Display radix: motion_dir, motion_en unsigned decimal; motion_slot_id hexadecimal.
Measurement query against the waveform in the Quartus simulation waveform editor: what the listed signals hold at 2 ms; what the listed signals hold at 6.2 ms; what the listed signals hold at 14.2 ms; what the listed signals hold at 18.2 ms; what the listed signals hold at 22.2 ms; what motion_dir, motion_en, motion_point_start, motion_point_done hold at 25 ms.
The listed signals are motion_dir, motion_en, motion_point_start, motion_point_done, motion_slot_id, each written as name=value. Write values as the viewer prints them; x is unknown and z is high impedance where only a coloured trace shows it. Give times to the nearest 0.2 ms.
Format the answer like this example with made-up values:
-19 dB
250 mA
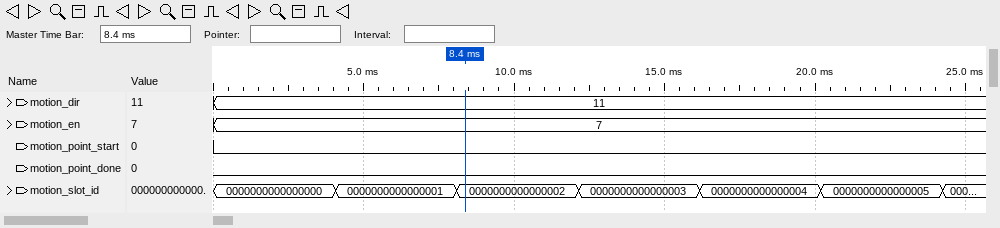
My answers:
motion_dir=11, motion_en=7, motion_point_start=0, motion_point_done=0, motion_slot_id=0000000000000000
motion_dir=11, motion_en=7, motion_point_start=0, motion_point_done=0, motion_slot_id=0000000000000001
motion_dir=11, motion_en=7, motion_point_start=0, motion_point_done=0, motion_slot_id=0000000000000003
motion_dir=11, motion_en=7, motion_point_start=0, motion_point_done=0, motion_slot_id=0000000000000004
motion_dir=11, motion_en=7, motion_point_start=0, motion_point_done=0, motion_slot_id=0000000000000005
motion_dir=11, motion_en=7, motion_point_start=0, motion_point_done=0
